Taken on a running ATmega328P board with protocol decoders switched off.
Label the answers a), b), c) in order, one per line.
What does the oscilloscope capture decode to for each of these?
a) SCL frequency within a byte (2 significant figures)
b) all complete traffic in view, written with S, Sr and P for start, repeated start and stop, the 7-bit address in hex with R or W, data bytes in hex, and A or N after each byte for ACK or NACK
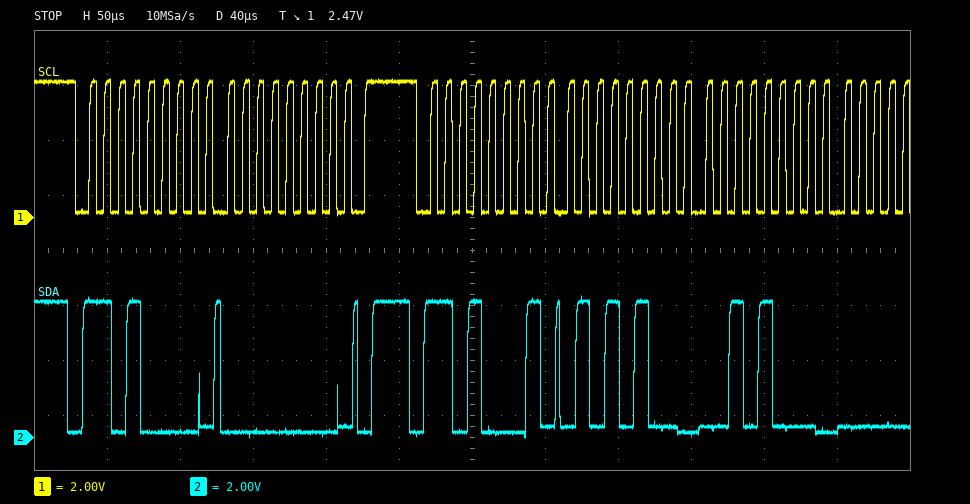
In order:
a) 100 kHz
b) S 68W A 00 A P S 68R A 54 A 28 A
